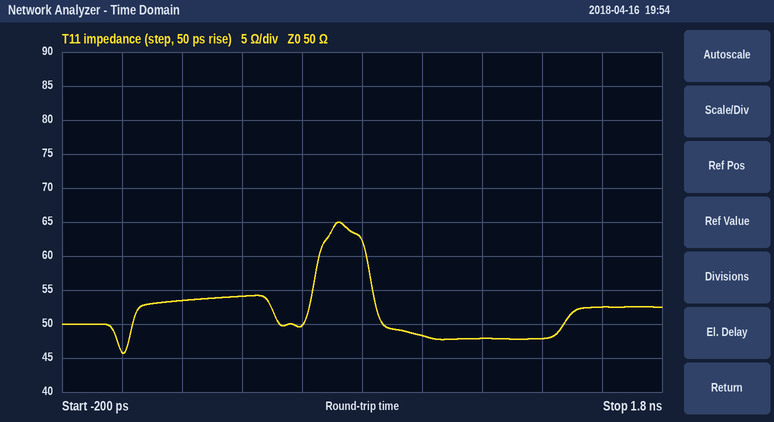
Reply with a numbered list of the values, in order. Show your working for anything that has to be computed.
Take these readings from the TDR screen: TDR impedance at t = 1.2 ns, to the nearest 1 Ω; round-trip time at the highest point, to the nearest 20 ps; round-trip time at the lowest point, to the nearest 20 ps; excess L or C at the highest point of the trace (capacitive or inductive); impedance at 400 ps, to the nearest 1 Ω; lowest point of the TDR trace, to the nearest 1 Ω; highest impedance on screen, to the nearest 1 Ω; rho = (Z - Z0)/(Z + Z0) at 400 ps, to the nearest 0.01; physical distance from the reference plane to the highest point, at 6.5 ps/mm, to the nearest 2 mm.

1. 48 Ω
2. 720 ps
3. 0 ps
4. inductive
5. 54 Ω
6. 46 Ω
7. 65 Ω
8. (54 − 50)/(54 + 50) ≈ +0.04
9. 720 ps / 2 / 6.5 ps/mm ≈ 55.4 mm, so 56 mm to the nearest 2 mm
